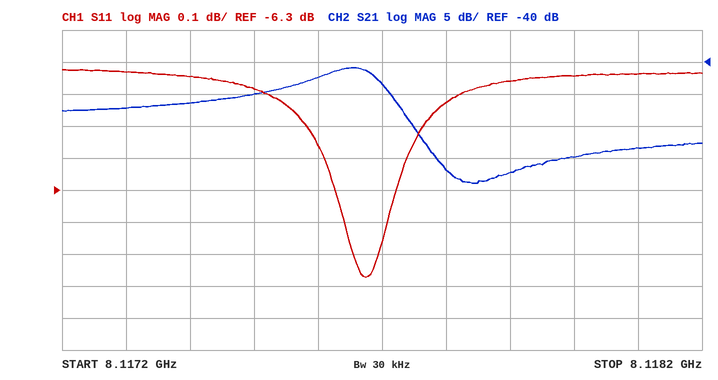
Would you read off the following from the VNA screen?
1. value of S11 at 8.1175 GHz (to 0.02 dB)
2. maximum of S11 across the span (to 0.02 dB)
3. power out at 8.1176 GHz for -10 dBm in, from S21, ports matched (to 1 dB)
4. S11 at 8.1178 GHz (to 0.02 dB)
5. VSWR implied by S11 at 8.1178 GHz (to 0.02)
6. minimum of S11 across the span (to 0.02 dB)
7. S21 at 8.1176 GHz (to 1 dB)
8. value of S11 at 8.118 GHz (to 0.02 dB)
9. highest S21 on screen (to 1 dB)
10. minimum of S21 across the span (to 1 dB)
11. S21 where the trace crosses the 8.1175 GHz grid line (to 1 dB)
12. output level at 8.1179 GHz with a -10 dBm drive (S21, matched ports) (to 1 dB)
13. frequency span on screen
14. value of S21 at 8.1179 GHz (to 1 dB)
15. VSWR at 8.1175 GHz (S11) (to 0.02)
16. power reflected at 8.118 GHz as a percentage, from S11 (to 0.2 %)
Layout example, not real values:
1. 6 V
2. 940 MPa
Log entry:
1. -5.98 dB
2. -5.92 dB
3. -52 dBm
4. -6.02 dB
5. 3.00
6. -6.58 dB
7. -42 dB
8. -5.94 dB
9. -41 dB
10. -59 dB
11. -45 dB
12. -67 dBm
13. 1 MHz
14. -57 dB
15. 3.02
16. 25.4 %
